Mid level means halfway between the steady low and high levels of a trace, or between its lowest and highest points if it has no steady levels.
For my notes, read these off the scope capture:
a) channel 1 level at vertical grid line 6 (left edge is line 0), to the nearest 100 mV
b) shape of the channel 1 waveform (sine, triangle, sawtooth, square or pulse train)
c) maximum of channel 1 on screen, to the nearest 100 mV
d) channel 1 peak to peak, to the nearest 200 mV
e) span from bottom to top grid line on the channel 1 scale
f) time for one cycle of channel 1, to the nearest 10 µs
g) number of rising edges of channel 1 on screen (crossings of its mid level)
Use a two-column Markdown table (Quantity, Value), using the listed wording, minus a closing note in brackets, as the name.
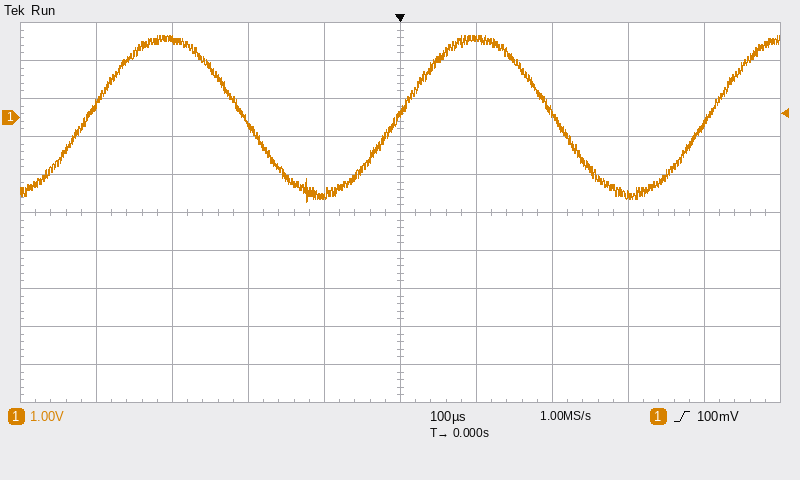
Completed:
| Quantity | Value |
|---|---|
| channel 1 level at vertical grid line 6 (left edge is line 0), to the nearest 100 mV | 2.1 V |
| shape of the channel 1 waveform | sine |
| maximum of channel 1 on screen, to the nearest 100 mV | 2.2 V |
| channel 1 peak to peak, to the nearest 200 mV | 4.4 V |
| span from bottom to top grid line on the channel 1 scale | 10 V |
| time for one cycle of channel 1, to the nearest 10 µs | 410 µs |
| number of rising edges of channel 1 on screen | 3 |
